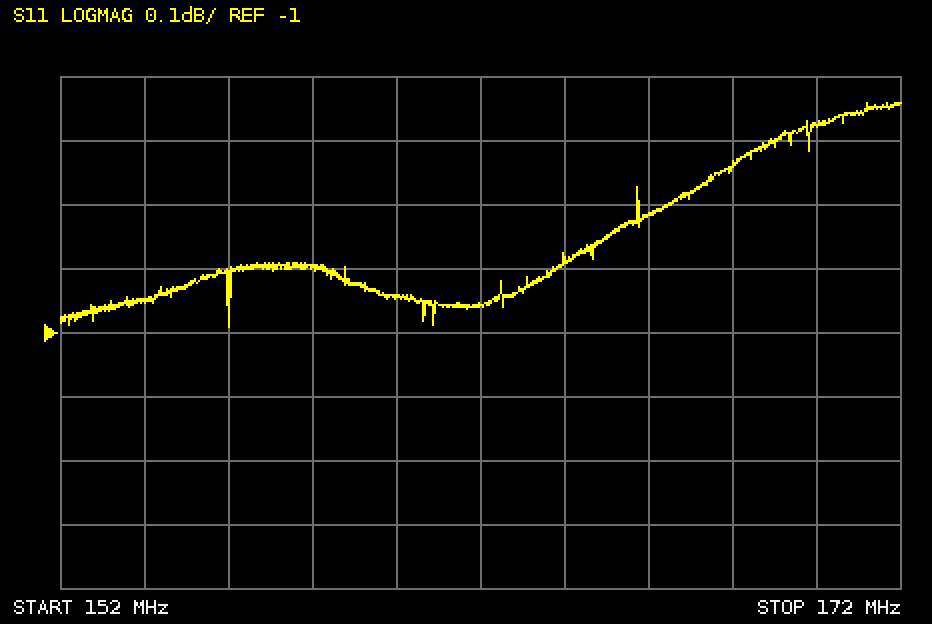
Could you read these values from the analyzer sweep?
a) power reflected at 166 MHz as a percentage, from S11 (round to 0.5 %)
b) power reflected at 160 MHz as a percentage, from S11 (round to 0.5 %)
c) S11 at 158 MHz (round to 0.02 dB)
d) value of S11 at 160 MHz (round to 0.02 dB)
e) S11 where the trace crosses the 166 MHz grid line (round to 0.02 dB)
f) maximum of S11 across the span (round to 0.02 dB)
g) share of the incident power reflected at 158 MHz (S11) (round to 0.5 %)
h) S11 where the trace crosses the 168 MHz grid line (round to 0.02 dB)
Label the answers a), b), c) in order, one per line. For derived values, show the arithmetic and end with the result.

a) 10^(-0.82/10) ≈ 82.8 %, so 83.0 % to the nearest 0.5 %
b) 10^(-0.94/10) ≈ 80.5 %
c) -0.90 dB
d) -0.94 dB
e) -0.82 dB
f) -0.64 dB
g) 10^(-0.9/10) ≈ 81.3 %, so 81.5 % to the nearest 0.5 %
h) -0.74 dB
